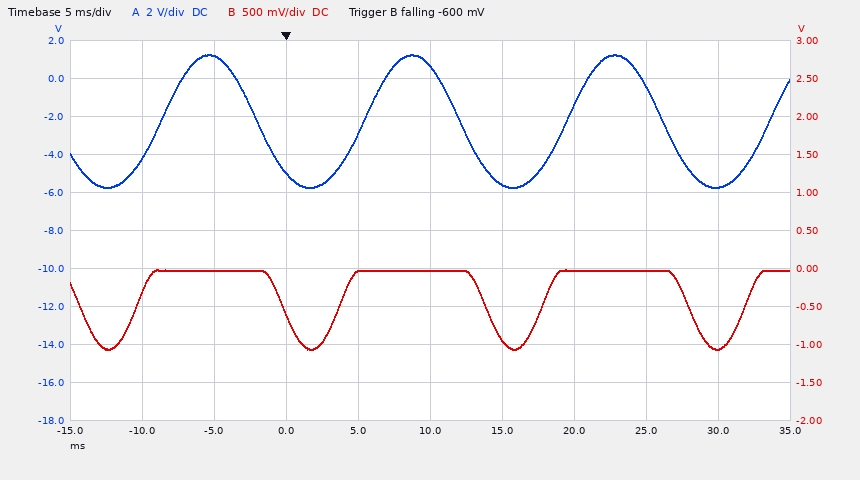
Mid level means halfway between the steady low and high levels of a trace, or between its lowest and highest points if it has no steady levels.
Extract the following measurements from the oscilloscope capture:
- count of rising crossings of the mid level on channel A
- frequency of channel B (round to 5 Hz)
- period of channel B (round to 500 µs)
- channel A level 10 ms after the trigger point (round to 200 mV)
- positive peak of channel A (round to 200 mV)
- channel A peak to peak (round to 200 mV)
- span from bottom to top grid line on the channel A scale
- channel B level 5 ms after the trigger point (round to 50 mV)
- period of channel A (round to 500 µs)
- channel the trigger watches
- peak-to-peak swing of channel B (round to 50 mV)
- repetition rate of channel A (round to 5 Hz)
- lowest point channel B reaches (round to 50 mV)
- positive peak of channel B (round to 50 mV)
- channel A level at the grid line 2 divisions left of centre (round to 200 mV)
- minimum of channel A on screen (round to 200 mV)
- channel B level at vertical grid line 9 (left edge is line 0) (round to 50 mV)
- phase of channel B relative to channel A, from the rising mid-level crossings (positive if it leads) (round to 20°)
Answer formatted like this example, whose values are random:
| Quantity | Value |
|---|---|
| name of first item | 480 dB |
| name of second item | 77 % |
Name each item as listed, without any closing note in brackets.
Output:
| Quantity | Value |
|---|---|
| count of rising crossings of the mid level on channel A | 4 |
| frequency of channel B | 70 Hz |
| period of channel B | 14.0 ms |
| channel A level 10 ms after the trigger point | 600 mV |
| positive peak of channel A | 1.2 V |
| channel A peak to peak | 7.0 V |
| span from bottom to top grid line on the channel A scale | 20 V |
| channel B level 5 ms after the trigger point | -50 mV |
| period of channel A | 14.0 ms |
| channel the trigger watches | channel B |
| peak-to-peak swing of channel B | 1.05 V |
| repetition rate of channel A | 70 Hz |
| lowest point channel B reaches | -1.05 V |
| positive peak of channel B | 0 mV |
| channel A level at the grid line 2 divisions left of centre | -5.0 V |
| minimum of channel A on screen | -5.8 V |
| channel B level at vertical grid line 9 (left edge is line 0) | -1.05 V |
| phase of channel B relative to channel A, from the rising mid-level crossings (positive if it leads) | +40° |
